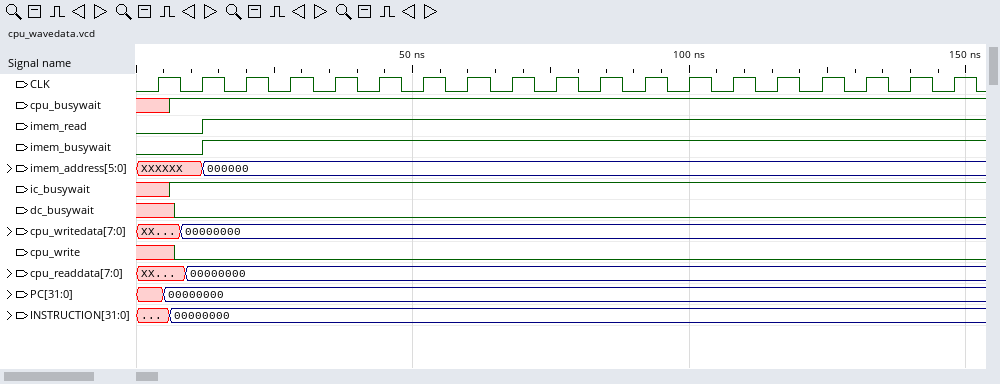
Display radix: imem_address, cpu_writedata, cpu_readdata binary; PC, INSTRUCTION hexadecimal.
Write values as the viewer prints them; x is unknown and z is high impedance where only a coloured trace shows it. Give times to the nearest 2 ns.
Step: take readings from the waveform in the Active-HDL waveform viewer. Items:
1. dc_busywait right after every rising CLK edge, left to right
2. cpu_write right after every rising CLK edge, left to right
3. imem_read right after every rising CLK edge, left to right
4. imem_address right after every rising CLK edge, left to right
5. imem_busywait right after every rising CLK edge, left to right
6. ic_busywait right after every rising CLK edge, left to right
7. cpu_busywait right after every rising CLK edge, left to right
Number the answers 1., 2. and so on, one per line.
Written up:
1. x 0 0 0 0 0 0 0 0 0 0 0 0 0 0 0 0 0 0
2. x 0 0 0 0 0 0 0 0 0 0 0 0 0 0 0 0 0 0
3. 0 1 1 1 1 1 1 1 1 1 1 1 1 1 1 1 1 1 1
4. XXXXXX, 000000, 000000, 000000, 000000, 000000, 000000, 000000, 000000, 000000, 000000, 000000, 000000, 000000, 000000, 000000, 000000, 000000, 000000
5. 0 1 1 1 1 1 1 1 1 1 1 1 1 1 1 1 1 1 1
6. x 1 1 1 1 1 1 1 1 1 1 1 1 1 1 1 1 1 1
7. x 1 1 1 1 1 1 1 1 1 1 1 1 1 1 1 1 1 1
